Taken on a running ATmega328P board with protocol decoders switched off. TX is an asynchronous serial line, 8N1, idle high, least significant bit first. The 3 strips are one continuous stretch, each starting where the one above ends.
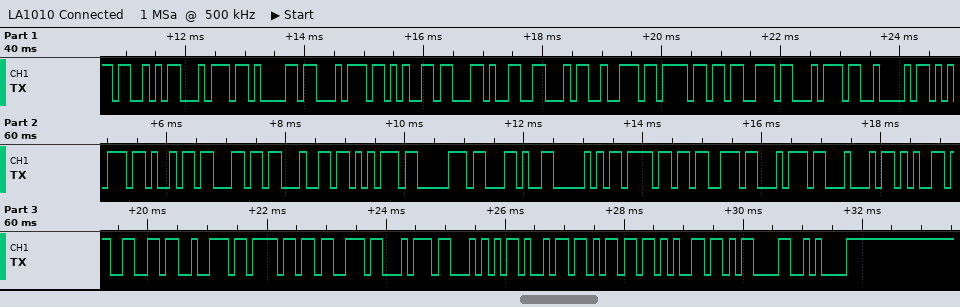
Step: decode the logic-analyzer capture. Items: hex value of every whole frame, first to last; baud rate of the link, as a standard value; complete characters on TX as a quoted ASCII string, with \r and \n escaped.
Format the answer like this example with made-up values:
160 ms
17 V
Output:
53 74 61 74 65 2C 46 72 6F 73 74 42 75 69 6C 64 75 70 2C 50 6F 73 74 44 65 66 72 6F 73 74 54 69 6D 65 0D 0A
9600 baud
"State,FrostBuildup,PostDefrostTime\r\n"
